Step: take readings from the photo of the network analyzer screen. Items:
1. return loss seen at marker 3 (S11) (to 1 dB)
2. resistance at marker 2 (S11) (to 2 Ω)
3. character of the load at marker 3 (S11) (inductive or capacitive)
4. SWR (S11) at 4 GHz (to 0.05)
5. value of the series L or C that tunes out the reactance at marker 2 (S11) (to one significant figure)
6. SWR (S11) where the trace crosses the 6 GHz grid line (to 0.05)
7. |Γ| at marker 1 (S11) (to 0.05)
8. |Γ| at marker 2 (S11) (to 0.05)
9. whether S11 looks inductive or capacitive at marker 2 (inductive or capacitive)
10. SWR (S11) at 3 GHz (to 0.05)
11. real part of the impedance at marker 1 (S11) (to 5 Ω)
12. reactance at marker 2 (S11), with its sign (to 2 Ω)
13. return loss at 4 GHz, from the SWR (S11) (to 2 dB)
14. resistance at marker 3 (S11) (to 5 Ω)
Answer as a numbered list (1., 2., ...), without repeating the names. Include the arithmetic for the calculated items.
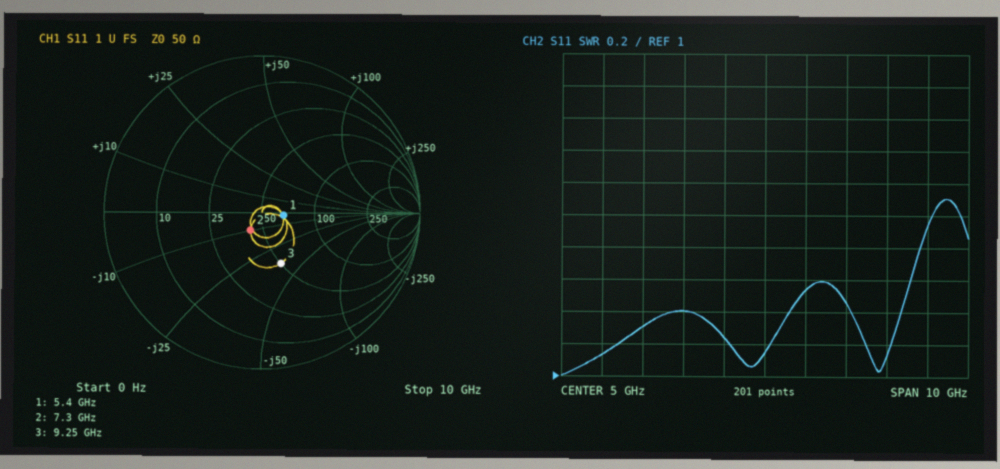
1. 9 dB
2. 42 Ω
3. capacitive
4. 1.25
5. L = 10 Ω/(2π × 7.3 GHz) ≈ 218 pH, so 200 pH to one significant figure
6. 1.55
7. 0.15
8. 0.15
9. capacitive
10. 1.40
11. 65 Ω
12. -10 Ω
13. −20 log10((1.25 − 1)/(1.25 + 1)) ≈ 19.1 dB, so 20 dB to the nearest 2 dB
14. 50 Ω
